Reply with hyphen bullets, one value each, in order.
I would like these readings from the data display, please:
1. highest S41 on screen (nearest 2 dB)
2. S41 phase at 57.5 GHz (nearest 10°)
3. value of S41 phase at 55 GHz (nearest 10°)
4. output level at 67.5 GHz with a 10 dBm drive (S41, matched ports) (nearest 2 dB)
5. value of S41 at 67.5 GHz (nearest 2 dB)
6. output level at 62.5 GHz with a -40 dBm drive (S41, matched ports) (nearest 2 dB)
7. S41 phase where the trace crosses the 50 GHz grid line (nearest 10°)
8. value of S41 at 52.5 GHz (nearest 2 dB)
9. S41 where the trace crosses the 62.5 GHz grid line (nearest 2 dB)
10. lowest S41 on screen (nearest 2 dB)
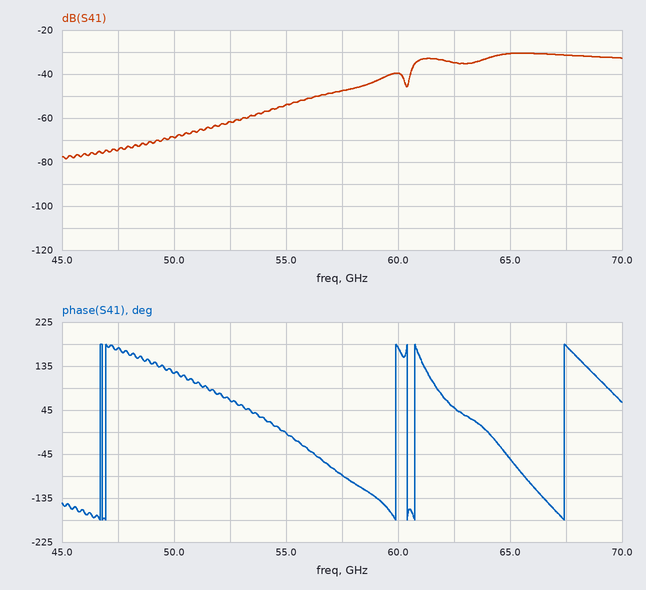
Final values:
- -30 dB
- -90°
- 0°
- -22 dBm
- -32 dB
- -74 dBm
- 120°
- -62 dB
- -34 dB
- -78 dB
